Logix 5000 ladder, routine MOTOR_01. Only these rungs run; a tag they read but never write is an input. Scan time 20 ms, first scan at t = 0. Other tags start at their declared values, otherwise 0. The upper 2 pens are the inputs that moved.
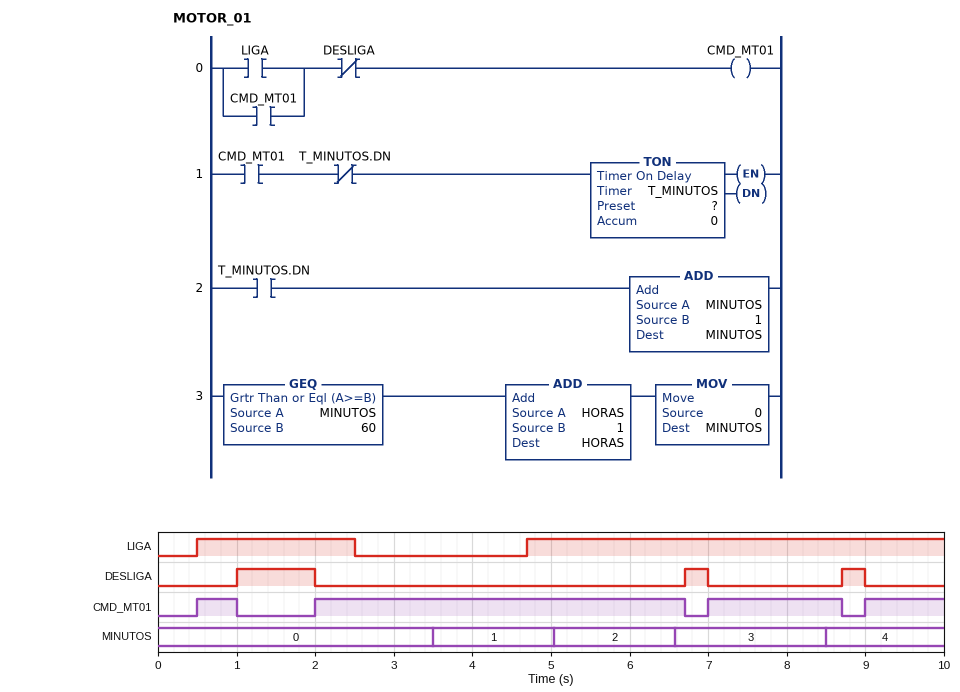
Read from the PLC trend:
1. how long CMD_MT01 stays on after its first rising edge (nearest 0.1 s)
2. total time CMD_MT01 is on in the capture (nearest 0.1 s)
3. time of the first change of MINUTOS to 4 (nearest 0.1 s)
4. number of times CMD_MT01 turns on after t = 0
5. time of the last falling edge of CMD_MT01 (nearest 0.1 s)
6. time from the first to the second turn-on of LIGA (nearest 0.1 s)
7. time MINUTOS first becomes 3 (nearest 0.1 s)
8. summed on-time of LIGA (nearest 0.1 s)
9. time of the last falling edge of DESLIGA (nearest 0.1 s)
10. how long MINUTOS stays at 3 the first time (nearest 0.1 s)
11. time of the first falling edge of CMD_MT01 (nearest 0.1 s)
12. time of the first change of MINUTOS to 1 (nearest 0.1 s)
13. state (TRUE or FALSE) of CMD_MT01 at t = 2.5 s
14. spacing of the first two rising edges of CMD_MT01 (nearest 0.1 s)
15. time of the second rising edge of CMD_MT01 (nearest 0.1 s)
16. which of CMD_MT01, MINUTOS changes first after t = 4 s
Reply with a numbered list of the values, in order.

1. 0.5 s
2. 7.9 s
3. 8.5 s
4. 4
5. 8.7 s
6. 4.2 s
7. 6.6 s
8. 7.3 s
9. 9.0 s
10. 1.9 s
11. 1.0 s
12. 3.5 s
13. TRUE
14. 1.5 s
15. 2.0 s
16. MINUTOS
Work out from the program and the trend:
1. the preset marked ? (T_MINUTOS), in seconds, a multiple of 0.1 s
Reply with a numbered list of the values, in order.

1. 1.5 s
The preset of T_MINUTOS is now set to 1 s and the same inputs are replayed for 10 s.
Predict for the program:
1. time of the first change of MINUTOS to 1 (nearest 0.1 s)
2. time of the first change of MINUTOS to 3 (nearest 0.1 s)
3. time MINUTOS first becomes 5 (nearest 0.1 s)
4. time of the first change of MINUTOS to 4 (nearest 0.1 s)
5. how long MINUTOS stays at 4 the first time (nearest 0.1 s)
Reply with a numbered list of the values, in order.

1. 3.0 s
2. 5.1 s
3. 8.0 s
4. 6.1 s
5. 1.9 s
